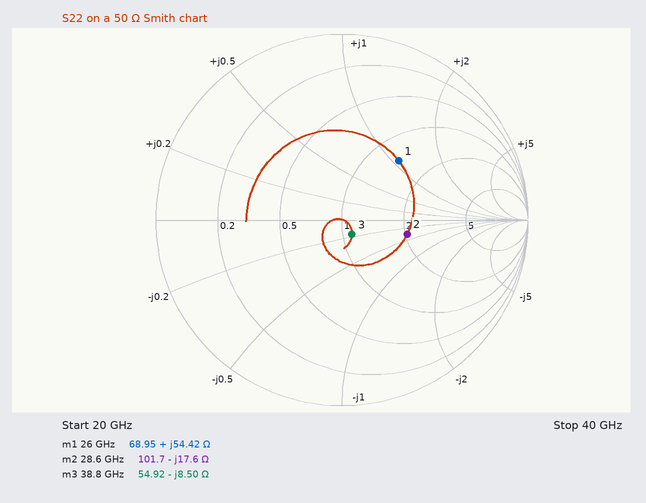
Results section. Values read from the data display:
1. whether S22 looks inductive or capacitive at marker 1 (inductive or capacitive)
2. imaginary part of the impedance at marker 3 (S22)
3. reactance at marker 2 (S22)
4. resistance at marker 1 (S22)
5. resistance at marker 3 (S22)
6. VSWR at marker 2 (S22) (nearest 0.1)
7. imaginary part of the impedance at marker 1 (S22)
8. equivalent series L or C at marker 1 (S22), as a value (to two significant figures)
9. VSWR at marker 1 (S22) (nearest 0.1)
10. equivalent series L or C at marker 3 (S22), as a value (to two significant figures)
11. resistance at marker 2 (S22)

inductive
-8.50 Ω
-17.6 Ω
68.95 Ω
54.92 Ω
2.1
+54.42 Ω
330 pH
2.6
480 fF
101.7 Ω
